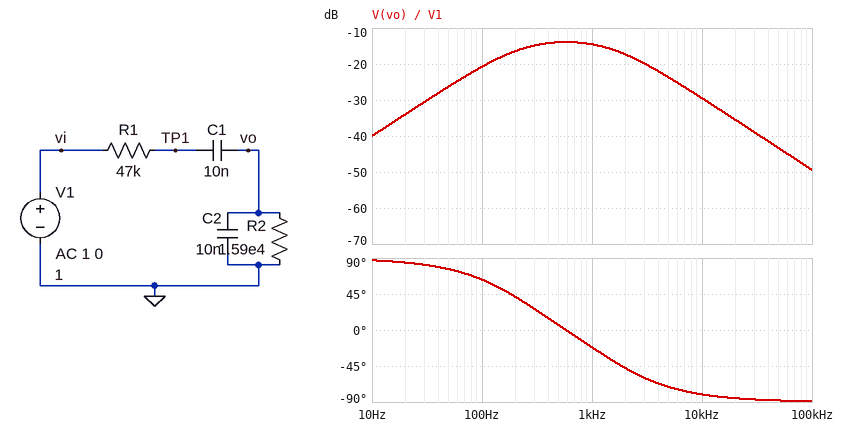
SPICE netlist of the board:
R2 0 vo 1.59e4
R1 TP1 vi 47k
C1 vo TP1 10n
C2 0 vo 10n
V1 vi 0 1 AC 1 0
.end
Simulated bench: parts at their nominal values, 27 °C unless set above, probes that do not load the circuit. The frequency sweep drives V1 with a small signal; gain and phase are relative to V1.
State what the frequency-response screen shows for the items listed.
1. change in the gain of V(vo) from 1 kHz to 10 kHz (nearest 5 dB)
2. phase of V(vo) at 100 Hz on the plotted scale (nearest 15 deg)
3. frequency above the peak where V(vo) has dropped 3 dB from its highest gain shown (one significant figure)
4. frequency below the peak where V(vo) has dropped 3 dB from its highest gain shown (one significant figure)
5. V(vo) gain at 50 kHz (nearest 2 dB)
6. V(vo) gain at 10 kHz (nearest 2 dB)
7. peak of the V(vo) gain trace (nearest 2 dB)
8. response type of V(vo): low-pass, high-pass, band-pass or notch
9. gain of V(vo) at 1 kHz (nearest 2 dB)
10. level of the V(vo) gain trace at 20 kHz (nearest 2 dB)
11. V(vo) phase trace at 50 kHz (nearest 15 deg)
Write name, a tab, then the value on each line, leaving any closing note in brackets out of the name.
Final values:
change in the gain of V(vo) from 1 kHz to 10 kHz	-15 dB
phase of V(vo) at 100 Hz on the plotted scale	60 deg
frequency above the peak where V(vo) has dropped 3 dB from its highest gain shown	2 kHz
frequency below the peak where V(vo) has dropped 3 dB from its highest gain shown	200 Hz
V(vo) gain at 50 kHz	-44 dB
V(vo) gain at 10 kHz	-30 dB
peak of the V(vo) gain trace	-14 dB
response type of V(vo): low-pass, high-pass, band-pass or notch	band-pass
gain of V(vo) at 1 kHz	-14 dB
level of the V(vo) gain trace at 20 kHz	-36 dB
V(vo) phase trace at 50 kHz	-90 deg
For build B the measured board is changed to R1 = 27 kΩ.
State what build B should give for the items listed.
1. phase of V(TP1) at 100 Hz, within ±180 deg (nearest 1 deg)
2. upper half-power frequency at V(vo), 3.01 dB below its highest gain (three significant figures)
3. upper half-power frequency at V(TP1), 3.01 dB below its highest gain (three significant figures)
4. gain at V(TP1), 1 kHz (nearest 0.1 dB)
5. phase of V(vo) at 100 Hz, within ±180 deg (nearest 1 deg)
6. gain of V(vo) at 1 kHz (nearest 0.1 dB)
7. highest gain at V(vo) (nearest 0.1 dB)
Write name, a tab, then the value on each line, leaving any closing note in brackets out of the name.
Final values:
phase of V(TP1) at 100 Hz, within ±180 deg	-9 deg
upper half-power frequency at V(vo), 3.01 dB below its highest gain	2.42 kHz
upper half-power frequency at V(TP1), 3.01 dB below its highest gain	561 Hz
gain at V(TP1), 1 kHz	-4.5 dB
phase of V(vo) at 100 Hz, within ±180 deg	69 deg
gain of V(vo) at 1 kHz	-11.5 dB
highest gain at V(vo)	-11.4 dB
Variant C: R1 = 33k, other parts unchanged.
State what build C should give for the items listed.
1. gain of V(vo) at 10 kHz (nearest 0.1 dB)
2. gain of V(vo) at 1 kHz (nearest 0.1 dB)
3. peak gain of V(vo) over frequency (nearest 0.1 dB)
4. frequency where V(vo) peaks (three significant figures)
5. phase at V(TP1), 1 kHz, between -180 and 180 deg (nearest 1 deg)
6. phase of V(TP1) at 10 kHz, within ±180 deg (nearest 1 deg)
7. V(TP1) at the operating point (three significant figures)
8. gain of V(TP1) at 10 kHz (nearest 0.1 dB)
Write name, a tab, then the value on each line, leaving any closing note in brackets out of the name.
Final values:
gain of V(vo) at 10 kHz	-26.5 dB
gain of V(vo) at 1 kHz	-12.5 dB
peak gain of V(vo) over frequency	-12.2 dB
frequency where V(vo) peaks	695 Hz
phase at V(TP1), 1 kHz, between -180 and 180 deg	-41 deg
phase of V(TP1) at 10 kHz, within ±180 deg	-82 deg
V(TP1) at the operating point	1.00 V
gain of V(TP1) at 10 kHz	-20.4 dB
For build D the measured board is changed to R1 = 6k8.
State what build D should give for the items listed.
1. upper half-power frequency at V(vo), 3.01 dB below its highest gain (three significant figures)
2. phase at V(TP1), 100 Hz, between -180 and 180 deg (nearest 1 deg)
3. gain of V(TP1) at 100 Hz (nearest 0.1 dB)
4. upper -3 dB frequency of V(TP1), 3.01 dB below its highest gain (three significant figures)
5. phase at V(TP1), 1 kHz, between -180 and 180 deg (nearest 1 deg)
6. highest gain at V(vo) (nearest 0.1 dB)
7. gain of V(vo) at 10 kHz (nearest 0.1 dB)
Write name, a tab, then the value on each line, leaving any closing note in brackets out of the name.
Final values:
upper half-power frequency at V(vo), 3.01 dB below its highest gain	6.07 kHz
phase at V(TP1), 100 Hz, between -180 and 180 deg	-2 deg
gain of V(TP1) at 100 Hz	0 dB
upper -3 dB frequency of V(TP1), 3.01 dB below its highest gain	4.07 kHz
phase at V(TP1), 1 kHz, between -180 and 180 deg	-13 deg
highest gain at V(vo)	-7.7 dB
gain of V(vo) at 10 kHz	-13.7 dB
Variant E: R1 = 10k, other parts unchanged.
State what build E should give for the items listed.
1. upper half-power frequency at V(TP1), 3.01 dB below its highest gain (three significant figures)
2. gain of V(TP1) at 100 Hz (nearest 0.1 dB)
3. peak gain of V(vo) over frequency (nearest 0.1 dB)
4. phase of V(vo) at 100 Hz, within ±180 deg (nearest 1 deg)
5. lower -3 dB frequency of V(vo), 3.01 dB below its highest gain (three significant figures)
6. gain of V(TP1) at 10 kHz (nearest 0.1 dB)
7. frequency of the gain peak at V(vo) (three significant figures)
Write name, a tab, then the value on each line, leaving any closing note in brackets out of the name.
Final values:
upper half-power frequency at V(TP1), 3.01 dB below its highest gain	2.52 kHz
gain of V(TP1) at 100 Hz	-0.1 dB
peak gain of V(vo) over frequency	-8.4 dB
phase of V(vo) at 100 Hz, within ±180 deg	75 deg
lower -3 dB frequency of V(vo), 3.01 dB below its highest gain	351 Hz
gain of V(TP1) at 10 kHz	-10.5 dB
frequency of the gain peak at V(vo)	1.26 kHz
